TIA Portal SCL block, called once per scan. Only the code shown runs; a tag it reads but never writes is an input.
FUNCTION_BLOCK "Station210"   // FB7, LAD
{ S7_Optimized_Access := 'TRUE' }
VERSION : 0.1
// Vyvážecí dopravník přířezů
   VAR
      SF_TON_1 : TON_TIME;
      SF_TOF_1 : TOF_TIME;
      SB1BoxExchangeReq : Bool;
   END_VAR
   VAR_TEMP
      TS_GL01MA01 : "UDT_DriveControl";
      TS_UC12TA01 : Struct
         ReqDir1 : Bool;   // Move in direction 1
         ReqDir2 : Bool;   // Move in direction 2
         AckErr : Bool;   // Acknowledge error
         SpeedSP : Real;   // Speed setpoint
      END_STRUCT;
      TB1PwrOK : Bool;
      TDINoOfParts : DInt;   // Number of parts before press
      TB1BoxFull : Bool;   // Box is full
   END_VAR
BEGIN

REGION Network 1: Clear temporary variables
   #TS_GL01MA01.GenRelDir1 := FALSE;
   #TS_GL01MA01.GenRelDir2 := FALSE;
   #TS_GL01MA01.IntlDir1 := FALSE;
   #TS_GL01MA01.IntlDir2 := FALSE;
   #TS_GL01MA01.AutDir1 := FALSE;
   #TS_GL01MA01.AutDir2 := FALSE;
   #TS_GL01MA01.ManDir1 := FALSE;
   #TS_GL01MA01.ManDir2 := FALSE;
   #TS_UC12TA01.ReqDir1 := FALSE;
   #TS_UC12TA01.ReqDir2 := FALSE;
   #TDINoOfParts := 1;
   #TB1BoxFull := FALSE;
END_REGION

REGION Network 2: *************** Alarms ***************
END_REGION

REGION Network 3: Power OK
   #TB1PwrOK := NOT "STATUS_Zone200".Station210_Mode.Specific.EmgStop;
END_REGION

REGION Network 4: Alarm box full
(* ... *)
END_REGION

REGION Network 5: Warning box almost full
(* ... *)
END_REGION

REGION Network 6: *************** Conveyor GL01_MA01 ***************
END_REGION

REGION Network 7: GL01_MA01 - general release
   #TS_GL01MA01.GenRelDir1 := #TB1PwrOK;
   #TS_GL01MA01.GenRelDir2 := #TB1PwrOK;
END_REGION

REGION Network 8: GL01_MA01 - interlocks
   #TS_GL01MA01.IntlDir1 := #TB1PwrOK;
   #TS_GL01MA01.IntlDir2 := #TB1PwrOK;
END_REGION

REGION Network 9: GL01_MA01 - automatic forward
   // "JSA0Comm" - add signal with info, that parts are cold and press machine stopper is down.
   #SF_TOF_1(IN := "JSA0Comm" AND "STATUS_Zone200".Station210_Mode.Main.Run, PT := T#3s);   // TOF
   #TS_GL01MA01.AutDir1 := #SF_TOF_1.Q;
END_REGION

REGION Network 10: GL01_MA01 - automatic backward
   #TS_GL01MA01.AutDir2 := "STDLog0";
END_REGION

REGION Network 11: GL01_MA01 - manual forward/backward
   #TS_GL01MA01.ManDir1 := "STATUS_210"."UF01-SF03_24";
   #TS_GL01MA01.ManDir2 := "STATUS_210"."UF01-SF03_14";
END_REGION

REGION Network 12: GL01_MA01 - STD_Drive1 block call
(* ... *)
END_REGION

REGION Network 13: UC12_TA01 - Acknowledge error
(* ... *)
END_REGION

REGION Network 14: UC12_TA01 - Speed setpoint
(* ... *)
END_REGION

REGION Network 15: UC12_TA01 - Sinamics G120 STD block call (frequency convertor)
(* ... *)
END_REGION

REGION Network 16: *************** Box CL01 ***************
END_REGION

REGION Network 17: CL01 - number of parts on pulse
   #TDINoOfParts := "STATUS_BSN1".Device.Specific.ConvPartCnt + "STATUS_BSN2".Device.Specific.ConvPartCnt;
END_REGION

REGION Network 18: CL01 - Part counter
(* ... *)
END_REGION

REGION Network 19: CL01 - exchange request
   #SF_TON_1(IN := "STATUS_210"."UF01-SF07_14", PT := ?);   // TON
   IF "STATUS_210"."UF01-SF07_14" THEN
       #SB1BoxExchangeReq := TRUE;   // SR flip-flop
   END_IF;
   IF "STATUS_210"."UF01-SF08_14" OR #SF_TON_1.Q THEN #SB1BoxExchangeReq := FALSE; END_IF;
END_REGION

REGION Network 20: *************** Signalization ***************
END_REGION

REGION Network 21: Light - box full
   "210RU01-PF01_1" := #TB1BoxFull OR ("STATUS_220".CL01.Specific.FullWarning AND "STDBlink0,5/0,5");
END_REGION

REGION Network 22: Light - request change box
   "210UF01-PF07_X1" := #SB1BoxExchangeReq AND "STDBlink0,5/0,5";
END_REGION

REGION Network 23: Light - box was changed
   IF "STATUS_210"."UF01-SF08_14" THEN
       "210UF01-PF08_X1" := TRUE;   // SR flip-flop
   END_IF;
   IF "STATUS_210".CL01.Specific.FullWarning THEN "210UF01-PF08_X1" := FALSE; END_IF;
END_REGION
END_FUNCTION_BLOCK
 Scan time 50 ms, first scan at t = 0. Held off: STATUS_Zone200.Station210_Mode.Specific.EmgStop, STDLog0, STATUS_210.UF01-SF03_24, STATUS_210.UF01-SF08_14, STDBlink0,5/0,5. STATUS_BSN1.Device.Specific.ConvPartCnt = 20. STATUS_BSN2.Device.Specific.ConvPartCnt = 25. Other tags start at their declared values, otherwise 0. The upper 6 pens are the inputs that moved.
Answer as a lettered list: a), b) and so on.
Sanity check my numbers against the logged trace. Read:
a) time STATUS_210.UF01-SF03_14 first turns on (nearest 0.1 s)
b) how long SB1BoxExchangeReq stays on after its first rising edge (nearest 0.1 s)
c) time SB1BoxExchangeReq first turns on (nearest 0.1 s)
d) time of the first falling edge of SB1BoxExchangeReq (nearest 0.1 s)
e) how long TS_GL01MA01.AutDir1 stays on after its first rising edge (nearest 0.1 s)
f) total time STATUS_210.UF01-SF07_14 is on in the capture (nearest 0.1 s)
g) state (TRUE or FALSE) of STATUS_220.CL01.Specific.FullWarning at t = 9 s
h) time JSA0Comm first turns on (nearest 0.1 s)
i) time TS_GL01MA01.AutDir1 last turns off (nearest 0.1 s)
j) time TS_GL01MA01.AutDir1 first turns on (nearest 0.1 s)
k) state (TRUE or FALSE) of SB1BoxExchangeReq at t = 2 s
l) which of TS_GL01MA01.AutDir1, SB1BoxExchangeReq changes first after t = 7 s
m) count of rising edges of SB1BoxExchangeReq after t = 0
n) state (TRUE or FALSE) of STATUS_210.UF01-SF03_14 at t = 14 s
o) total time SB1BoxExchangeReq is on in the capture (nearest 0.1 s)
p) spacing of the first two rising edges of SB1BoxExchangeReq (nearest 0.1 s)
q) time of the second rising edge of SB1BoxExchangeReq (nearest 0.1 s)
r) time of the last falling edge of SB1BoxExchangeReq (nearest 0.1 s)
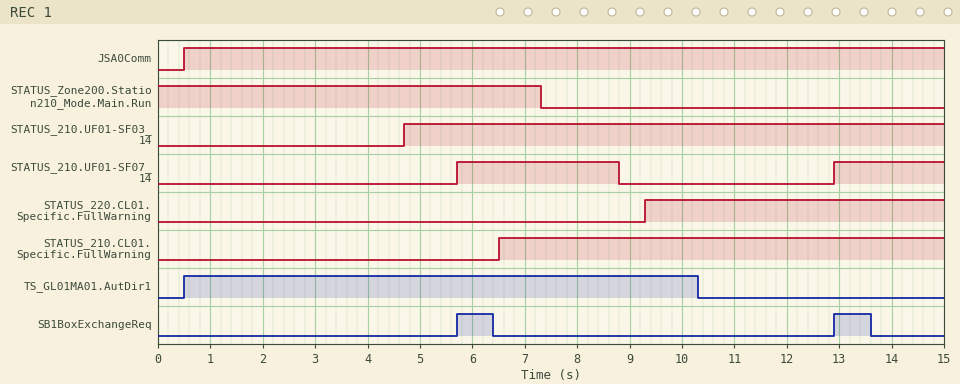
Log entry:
a) 4.7 s
b) 0.7 s
c) 5.7 s
d) 6.4 s
e) 9.8 s
f) 5.2 s
g) FALSE
h) 0.5 s
i) 10.3 s
j) 0.5 s
k) FALSE
l) TS_GL01MA01.AutDir1
m) 2
n) TRUE
o) 1.4 s
p) 7.2 s
q) 12.9 s
r) 13.6 s
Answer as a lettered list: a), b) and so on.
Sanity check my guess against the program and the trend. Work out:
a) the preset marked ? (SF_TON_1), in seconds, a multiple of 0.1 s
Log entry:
a) 0.7 s
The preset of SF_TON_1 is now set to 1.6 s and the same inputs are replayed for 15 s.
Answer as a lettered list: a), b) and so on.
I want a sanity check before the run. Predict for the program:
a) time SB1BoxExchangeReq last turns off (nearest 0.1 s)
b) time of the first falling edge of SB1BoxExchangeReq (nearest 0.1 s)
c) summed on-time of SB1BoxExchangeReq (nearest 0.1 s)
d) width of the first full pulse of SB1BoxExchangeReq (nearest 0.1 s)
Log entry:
a) 14.5 s
b) 7.3 s
c) 3.2 s
d) 1.6 s
